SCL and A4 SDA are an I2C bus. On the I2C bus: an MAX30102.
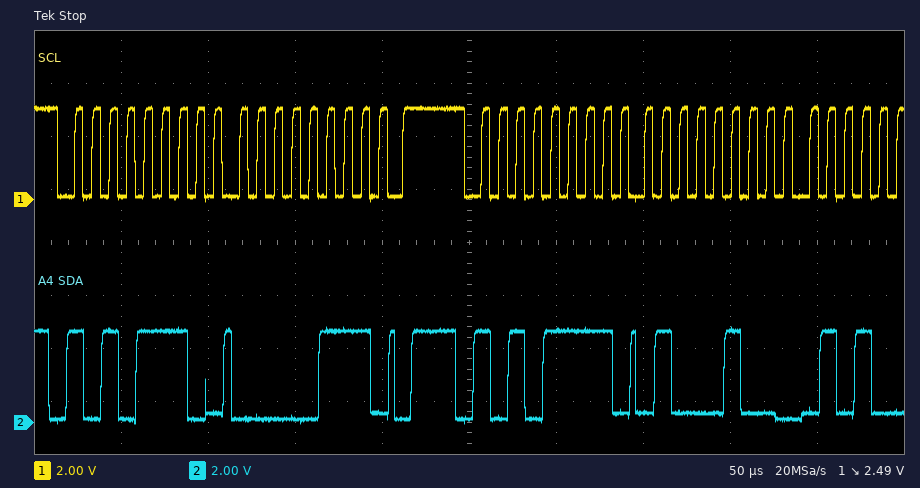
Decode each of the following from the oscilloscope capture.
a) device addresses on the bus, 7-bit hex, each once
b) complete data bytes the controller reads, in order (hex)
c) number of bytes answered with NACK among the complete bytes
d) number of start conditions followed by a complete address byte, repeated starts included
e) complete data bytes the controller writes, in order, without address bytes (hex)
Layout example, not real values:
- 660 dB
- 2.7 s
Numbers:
- 0x57
- 44
- 0
- 2
- 07
